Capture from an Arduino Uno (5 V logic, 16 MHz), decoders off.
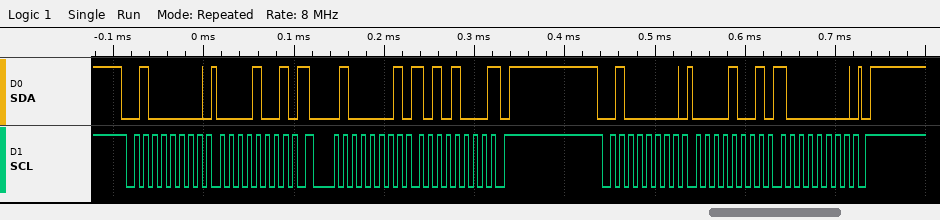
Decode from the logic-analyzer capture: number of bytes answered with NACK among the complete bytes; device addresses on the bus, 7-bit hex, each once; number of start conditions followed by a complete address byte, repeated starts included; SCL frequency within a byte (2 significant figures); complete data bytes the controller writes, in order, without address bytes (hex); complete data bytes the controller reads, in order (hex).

1
0x20
3
100 kHz
09 09 80
A8
